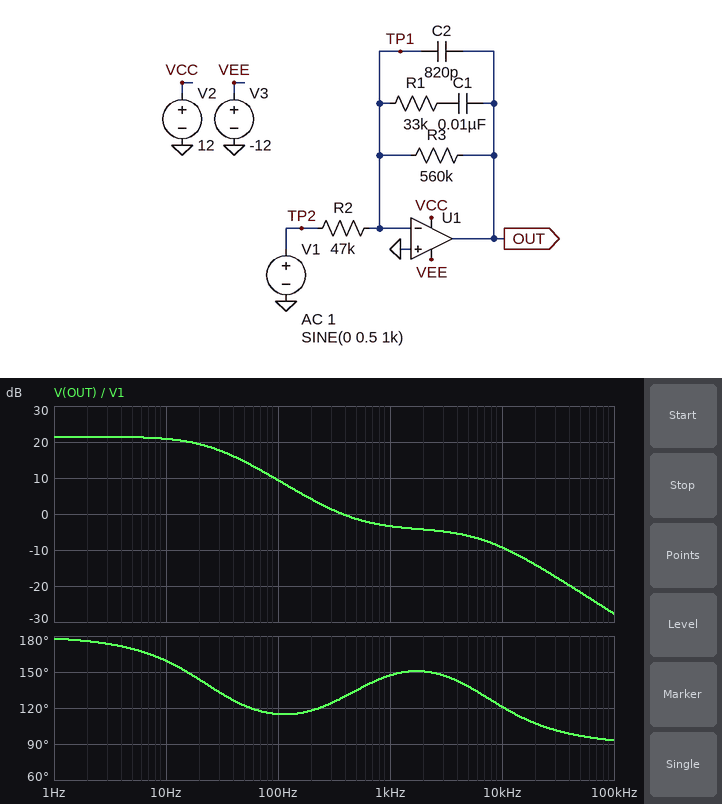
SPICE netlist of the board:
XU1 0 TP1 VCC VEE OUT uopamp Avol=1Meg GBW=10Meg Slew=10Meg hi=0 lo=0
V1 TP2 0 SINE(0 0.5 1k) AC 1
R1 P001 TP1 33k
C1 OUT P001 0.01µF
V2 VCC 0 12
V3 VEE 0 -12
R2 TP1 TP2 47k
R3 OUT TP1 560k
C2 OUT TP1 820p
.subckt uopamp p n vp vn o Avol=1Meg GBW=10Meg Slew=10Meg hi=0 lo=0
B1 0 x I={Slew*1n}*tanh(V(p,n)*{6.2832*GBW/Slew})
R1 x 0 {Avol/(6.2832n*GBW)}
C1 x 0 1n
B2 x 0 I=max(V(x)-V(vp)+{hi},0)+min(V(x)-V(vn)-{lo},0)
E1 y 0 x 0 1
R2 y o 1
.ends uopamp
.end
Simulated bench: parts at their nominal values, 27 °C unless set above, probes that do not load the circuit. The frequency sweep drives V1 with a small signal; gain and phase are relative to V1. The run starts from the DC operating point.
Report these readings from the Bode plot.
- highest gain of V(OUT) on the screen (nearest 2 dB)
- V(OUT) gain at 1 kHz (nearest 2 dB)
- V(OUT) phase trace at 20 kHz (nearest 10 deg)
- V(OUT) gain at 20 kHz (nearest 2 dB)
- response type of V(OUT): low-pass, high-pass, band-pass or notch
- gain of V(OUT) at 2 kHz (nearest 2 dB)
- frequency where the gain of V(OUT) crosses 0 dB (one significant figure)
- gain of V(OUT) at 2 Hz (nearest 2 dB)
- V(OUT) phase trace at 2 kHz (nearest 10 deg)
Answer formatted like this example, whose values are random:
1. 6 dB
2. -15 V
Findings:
1. 22 dB
2. -4 dB
3. 110 deg
4. -14 dB
5. low-pass
6. -4 dB
7. 400 Hz
8. 22 dB
9. 150 deg
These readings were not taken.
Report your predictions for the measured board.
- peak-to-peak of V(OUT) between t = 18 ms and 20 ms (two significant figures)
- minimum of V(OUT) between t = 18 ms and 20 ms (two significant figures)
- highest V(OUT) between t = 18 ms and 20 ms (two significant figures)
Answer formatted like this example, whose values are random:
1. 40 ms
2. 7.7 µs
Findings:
1. 680 mV
2. -350 mV
3. 330 mV
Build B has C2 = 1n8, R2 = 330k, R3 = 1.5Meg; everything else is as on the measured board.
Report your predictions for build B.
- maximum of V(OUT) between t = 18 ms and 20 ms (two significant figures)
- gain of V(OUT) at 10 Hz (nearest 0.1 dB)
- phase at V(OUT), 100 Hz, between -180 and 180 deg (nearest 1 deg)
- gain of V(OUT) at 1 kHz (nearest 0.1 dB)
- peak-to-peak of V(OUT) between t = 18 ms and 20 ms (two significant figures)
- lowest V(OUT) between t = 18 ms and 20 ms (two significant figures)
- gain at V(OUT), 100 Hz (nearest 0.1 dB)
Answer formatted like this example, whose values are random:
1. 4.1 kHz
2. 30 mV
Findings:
1. 38 mV
2. 9.6 dB
3. 105 deg
4. -21.1 dB
5. 89 mV
6. -51 mV
7. -7.8 dB
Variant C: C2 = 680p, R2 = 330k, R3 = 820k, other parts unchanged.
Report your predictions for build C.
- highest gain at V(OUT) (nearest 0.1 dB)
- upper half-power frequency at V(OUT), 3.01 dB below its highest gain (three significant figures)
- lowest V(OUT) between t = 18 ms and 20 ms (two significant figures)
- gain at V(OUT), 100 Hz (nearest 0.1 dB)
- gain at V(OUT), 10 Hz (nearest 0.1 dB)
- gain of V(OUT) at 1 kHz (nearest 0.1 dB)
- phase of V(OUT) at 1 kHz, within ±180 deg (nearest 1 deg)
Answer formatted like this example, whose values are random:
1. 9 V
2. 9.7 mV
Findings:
1. 7.9 dB
2. 17.6 Hz
3. -53 mV
4. -7.2 dB
5. 6.7 dB
6. -20.0 dB
7. 148 deg
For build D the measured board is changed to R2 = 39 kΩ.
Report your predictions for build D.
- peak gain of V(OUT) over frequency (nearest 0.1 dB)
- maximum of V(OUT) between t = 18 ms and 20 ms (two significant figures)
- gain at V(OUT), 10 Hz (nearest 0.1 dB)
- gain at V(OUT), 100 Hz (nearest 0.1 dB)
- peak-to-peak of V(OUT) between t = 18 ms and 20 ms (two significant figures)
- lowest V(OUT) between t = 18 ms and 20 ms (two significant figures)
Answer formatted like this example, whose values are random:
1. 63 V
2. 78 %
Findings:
1. 23.1 dB
2. 400 mV
3. 22.5 dB
4. 11.0 dB
5. 820 mV
6. -420 mV
